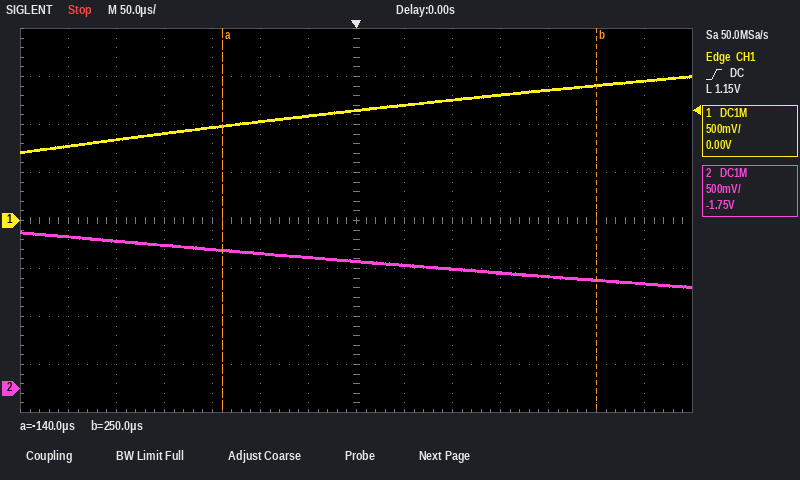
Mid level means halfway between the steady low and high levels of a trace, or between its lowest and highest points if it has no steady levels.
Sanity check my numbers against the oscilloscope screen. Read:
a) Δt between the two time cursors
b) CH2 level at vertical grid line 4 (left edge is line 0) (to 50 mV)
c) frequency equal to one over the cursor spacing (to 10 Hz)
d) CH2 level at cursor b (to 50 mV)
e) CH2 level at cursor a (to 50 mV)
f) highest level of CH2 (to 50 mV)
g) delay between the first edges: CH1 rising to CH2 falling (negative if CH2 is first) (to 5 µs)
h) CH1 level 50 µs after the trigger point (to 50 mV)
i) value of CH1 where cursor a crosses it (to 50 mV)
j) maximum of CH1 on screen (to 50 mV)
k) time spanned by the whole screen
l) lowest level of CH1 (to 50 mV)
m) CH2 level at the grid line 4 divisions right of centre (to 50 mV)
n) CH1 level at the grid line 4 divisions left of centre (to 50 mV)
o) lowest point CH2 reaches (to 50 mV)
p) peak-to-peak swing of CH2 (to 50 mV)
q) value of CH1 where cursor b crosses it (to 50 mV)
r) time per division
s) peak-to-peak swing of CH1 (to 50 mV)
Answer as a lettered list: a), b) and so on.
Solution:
a) 390 µs
b) 1.45 V
c) 2.56 kHz
d) 1.15 V
e) 1.45 V
f) 1.65 V
g) +20 µs
h) 1.20 V
i) 1.00 V
j) 1.50 V
k) 700 µs
l) 700 mV
m) 1.15 V
n) 900 mV
o) 1.05 V
p) 600 mV
q) 1.40 V
r) 50 µs
s) 800 mV
